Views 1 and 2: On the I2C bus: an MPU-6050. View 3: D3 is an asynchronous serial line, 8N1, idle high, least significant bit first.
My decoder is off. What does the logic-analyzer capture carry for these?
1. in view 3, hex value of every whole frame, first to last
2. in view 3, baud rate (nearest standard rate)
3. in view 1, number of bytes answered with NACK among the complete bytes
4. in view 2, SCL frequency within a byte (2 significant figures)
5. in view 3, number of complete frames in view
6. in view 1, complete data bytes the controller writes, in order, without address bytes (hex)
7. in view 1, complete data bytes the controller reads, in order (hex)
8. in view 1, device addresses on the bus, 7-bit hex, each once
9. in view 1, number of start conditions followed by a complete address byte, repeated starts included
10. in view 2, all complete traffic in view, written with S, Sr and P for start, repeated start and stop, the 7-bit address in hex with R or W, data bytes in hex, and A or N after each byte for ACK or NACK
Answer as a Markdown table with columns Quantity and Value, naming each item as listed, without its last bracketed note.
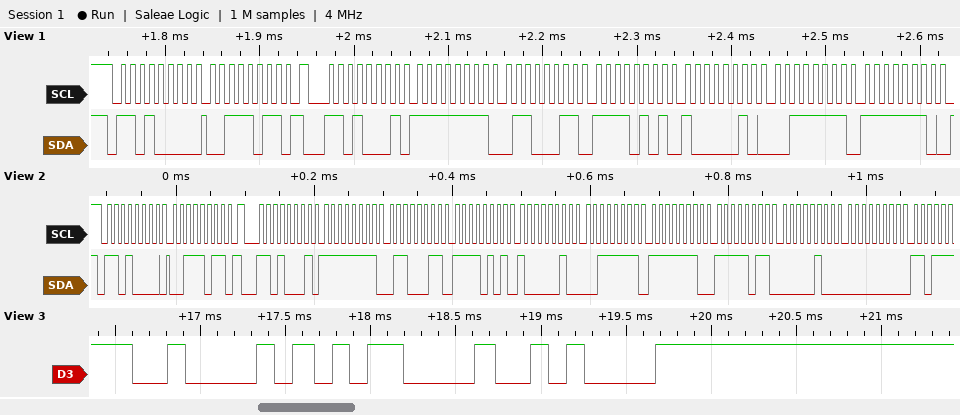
| Quantity | Value |
|---|---|
| in view 3, hex value of every whole frame, first to last | 42 0D 0A |
| in view 3, baud rate | 9600 baud |
| in view 1, number of bytes answered with NACK among the complete bytes | 0 |
| in view 2, SCL frequency within a byte | 100 kHz |
| in view 3, number of complete frames in view | 3 |
| in view 1, complete data bytes the controller writes, in order, without address bytes | 3B |
| in view 1, complete data bytes the controller reads, in order | FF 63 F5 82 3F FE |
| in view 1, device addresses on the bus, 7-bit hex, each once | 0x68 |
| in view 1, number of start conditions followed by a complete address byte, repeated starts included | 2 |
| in view 2, all complete traffic in view, written with S, Sr and P for start, repeated start and stop, the 7-bit address in hex with R or W, data bytes in hex, and A or N after each byte for ACK or NACK | S 68W A 3B A Sr 68R A FF A 63 A F5 A 82 A 3F A FE A FB A 04 A 00 A |
